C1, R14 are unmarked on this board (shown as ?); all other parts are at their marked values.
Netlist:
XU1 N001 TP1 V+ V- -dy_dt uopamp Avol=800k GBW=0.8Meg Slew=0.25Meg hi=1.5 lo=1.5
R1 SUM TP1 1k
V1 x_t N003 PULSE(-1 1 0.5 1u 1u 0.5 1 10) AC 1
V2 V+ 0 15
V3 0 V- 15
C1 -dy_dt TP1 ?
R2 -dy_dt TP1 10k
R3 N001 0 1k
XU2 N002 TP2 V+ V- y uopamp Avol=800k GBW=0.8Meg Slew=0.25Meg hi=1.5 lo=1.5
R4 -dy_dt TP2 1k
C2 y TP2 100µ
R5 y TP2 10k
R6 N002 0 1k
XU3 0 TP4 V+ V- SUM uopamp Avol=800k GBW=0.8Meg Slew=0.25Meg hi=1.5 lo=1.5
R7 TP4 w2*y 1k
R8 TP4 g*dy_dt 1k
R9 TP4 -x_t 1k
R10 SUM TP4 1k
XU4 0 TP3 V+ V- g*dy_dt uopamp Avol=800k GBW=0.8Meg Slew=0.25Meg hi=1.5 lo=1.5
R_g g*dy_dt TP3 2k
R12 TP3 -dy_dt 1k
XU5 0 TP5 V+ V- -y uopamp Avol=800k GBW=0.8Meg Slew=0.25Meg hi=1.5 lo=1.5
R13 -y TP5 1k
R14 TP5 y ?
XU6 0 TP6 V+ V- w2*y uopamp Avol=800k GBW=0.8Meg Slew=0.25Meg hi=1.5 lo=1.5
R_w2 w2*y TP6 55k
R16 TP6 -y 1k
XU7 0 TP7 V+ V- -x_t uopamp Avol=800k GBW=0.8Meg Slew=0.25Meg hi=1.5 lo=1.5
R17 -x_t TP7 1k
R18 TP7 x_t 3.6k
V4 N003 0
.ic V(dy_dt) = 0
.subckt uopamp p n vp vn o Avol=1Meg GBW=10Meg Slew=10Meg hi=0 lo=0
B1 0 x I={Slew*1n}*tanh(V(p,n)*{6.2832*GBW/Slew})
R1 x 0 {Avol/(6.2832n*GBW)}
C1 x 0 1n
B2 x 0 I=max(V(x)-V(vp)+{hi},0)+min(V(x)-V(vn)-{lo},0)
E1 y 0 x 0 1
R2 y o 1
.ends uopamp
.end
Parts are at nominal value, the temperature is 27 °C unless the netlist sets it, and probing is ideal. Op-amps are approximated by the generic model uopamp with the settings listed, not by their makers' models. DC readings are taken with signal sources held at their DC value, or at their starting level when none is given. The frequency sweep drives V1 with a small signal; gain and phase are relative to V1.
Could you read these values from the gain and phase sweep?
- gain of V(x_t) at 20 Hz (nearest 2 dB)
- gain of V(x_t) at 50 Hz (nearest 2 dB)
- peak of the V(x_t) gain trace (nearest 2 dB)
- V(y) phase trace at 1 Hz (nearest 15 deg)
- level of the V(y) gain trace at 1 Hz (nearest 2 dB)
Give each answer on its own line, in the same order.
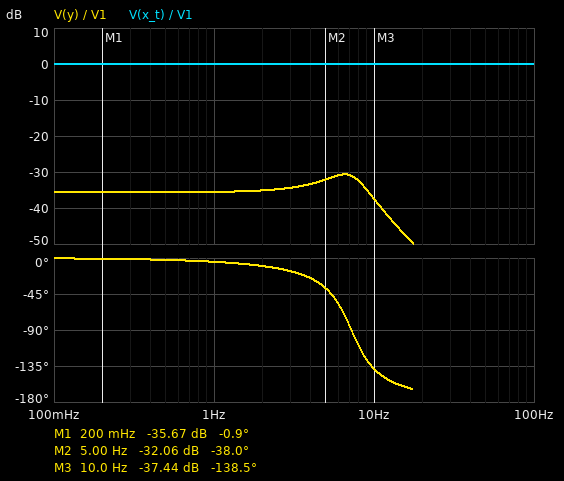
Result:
0 dB
0 dB
0 dB
0 deg
-36 dB
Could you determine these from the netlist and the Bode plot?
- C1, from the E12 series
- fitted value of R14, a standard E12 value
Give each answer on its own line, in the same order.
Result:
82 µF
3.3 kΩ
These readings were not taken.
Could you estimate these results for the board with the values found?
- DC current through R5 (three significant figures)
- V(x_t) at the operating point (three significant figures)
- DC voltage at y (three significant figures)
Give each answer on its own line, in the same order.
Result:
1.65 µA
-1.00 V
-16.5 mV
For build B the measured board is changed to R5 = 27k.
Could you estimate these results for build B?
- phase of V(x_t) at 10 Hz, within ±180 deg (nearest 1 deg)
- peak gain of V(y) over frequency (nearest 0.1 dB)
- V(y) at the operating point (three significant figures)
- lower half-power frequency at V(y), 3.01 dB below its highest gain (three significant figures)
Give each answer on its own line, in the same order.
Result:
0 deg
-30.4 dB
-16.6 mV
3.84 Hz
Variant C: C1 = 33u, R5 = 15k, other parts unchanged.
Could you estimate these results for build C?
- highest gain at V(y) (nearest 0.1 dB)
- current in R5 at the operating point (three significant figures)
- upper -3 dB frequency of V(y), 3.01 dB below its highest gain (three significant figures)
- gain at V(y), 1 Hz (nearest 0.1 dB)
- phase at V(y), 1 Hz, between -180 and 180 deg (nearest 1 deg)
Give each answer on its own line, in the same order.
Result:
-33.7 dB
1.10 µA
13.4 Hz
-35.6 dB
-5 deg
